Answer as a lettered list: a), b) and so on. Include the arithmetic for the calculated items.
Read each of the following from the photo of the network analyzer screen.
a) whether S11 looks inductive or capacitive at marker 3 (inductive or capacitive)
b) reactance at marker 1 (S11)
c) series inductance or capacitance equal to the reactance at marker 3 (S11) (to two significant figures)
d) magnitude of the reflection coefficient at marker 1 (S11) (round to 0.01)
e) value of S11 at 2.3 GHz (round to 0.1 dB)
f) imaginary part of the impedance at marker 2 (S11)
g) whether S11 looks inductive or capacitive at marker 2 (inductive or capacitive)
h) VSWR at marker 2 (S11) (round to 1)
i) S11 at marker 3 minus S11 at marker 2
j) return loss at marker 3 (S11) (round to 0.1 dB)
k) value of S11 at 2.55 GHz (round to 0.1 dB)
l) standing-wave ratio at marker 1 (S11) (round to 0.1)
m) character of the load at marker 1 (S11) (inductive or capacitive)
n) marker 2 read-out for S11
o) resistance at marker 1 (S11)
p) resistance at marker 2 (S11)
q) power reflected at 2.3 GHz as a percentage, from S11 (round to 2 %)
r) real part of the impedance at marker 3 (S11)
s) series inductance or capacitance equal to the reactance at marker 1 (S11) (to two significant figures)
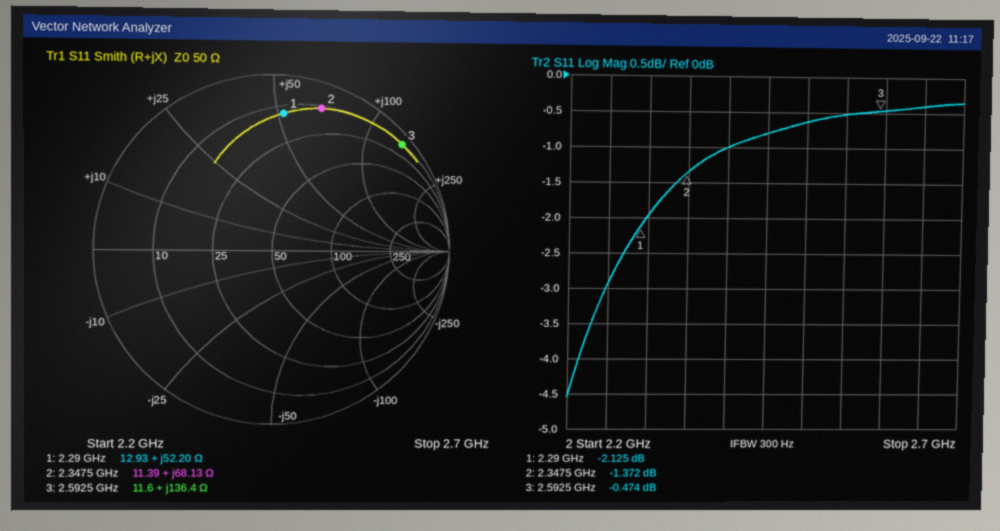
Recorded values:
a) inductive
b) +52.20 Ω
c) L = 136.4 Ω/(2π × 2.5925 GHz) ≈ 8.4 nH
d) 10^(-2.125/20) ≈ 0.78
e) -2.0 dB
f) +68.13 Ω
g) inductive
h) 13
i) -0.474 − (-1.372) = 0.898 dB
j) 0.5 dB
k) -0.5 dB
l) 8.2
m) inductive
n) -1.372 dB
o) 12.93 Ω
p) 11.39 Ω
q) 10^(-2/10) ≈ 63.1 %, so 64 % to the nearest 2 %
r) 11.6 Ω
s) L = 52.2 Ω/(2π × 2.29 GHz) ≈ 3.6 nH
